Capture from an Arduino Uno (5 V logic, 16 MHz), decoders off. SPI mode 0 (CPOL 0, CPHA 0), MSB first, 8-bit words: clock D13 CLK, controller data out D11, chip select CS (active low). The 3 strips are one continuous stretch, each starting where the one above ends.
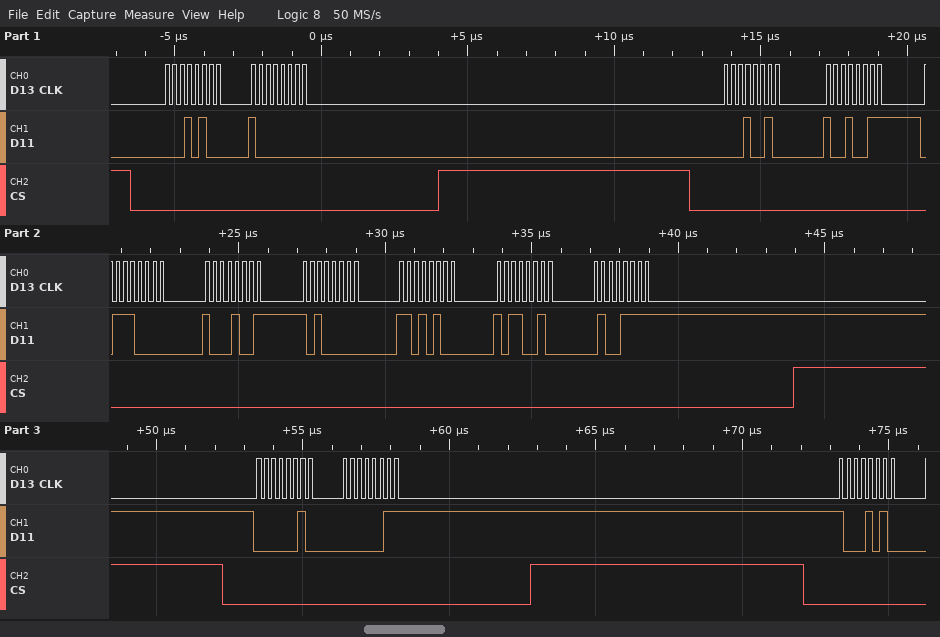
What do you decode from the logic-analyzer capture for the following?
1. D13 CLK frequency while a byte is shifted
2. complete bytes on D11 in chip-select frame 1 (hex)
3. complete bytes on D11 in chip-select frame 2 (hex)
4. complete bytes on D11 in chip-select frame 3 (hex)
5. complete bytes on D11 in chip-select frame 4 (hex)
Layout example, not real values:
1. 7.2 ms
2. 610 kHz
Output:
1. 4 MHz
2. 0x14 0x80
3. 0x12 0x93 0x70 0x89 0xA0 0xD4 0xB2 0x4F
4. 0x02 0x03
5. 0x8A
